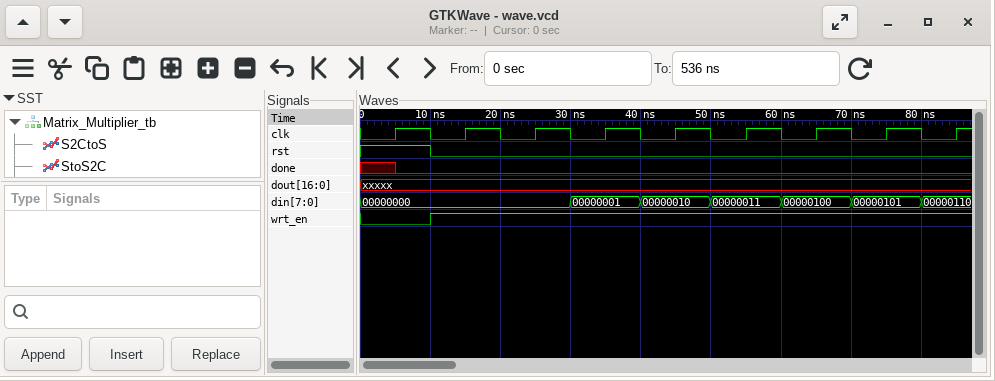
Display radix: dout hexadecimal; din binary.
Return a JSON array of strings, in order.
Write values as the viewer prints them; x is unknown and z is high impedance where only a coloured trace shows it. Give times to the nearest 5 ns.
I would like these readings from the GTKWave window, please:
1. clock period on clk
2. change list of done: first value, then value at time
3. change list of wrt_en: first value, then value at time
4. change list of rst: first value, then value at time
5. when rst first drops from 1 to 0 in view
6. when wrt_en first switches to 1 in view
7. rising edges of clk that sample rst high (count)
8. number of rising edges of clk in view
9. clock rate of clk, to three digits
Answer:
["10 ns", "x, 0 at 5 ns", "0, 1 at 10 ns", "1, 0 at 10 ns", "10 ns", "10 ns", "1", "9", "100 MHz"]
